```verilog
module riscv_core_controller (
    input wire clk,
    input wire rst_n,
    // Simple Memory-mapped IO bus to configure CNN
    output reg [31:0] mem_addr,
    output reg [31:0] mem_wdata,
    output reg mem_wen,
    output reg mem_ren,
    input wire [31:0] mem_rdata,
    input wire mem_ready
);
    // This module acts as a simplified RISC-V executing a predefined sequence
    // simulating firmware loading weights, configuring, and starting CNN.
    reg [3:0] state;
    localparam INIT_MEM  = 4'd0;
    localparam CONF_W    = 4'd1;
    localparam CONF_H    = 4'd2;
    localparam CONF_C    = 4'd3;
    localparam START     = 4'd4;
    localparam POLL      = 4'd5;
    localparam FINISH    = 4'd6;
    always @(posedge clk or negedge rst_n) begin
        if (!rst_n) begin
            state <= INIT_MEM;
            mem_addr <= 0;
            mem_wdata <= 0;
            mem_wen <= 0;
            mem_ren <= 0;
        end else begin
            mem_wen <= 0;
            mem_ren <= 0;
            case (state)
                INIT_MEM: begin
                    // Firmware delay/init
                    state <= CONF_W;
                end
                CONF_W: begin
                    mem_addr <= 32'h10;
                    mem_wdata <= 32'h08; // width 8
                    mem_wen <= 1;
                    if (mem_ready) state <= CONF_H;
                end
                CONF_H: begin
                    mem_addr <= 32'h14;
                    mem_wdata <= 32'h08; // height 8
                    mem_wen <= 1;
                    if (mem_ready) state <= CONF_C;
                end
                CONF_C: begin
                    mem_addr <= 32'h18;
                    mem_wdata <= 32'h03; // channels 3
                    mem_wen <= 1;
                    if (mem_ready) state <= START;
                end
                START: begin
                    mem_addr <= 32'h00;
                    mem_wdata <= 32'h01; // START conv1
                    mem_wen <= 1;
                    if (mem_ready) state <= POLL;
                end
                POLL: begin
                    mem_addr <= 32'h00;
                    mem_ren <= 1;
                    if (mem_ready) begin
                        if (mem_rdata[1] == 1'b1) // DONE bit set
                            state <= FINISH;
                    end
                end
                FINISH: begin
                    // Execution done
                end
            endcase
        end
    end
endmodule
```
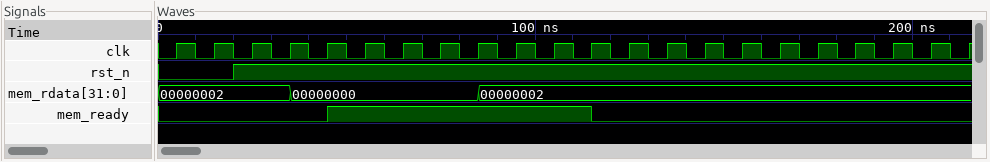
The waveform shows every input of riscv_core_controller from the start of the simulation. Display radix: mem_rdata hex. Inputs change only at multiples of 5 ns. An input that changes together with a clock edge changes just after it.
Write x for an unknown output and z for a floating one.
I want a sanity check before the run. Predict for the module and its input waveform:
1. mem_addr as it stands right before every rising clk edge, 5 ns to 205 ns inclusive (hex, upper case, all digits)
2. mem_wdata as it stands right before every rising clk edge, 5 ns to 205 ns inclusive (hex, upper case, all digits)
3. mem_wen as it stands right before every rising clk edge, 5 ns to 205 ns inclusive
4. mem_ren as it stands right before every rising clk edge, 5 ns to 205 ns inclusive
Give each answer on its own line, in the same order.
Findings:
00000000, 00000000, 00000000, 00000000, 00000010, 00000010, 00000010, 00000014, 00000018, 00000000, 00000000, 00000000, 00000000, 00000000, 00000000, 00000000, 00000000, 00000000, 00000000, 00000000, 00000000
00000000, 00000000, 00000000, 00000000, 00000008, 00000008, 00000008, 00000008, 00000003, 00000001, 00000001, 00000001, 00000001, 00000001, 00000001, 00000001, 00000001, 00000001, 00000001, 00000001, 00000001
0 0 0 0 1 1 1 1 1 1 0 0 0 0 0 0 0 0 0 0 0
0 0 0 0 0 0 0 0 0 0 1 0 0 0 0 0 0 0 0 0 0
